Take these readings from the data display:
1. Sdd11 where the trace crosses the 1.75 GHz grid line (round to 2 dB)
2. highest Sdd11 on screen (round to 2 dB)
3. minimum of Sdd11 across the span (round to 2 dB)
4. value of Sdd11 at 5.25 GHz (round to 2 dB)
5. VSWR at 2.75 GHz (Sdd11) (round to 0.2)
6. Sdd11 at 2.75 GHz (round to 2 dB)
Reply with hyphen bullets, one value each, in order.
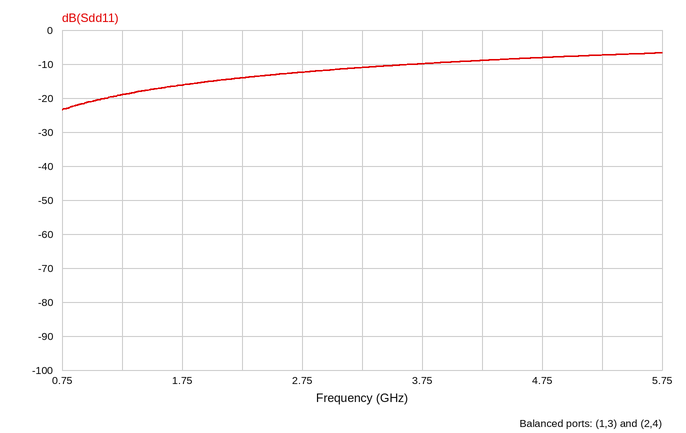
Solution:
- -16 dB
- -6 dB
- -24 dB
- -8 dB
- 1.6
- -12 dB
